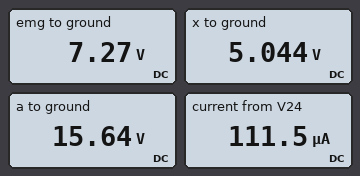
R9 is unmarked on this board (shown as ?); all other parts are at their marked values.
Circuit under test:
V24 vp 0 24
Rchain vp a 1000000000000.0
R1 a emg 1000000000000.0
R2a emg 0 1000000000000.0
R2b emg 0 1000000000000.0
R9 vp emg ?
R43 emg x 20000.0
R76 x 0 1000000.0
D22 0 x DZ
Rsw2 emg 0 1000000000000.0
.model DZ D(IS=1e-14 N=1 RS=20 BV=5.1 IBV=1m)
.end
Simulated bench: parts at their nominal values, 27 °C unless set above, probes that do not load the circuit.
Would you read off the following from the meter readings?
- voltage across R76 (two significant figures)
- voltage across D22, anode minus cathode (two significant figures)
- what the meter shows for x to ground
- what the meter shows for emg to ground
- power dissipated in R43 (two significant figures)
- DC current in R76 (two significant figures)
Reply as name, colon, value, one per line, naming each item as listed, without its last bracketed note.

voltage across R76: 5.0 V
voltage across D22, anode minus cathode: -5.0 V
what the meter shows for x to ground: 5.044 V
what the meter shows for emg to ground: 7.27 V
power dissipated in R43: 250 µW
DC current in R76: 5.0 µA
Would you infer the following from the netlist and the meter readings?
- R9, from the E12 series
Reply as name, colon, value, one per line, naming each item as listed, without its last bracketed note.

R9, from the E12 series: 150 kΩ
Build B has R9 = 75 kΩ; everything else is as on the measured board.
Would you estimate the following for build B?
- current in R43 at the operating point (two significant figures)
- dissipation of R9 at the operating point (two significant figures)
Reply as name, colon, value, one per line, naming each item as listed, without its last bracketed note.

current in R43 at the operating point: 200 µA
dissipation of R9 at the operating point: 3.0 mW
